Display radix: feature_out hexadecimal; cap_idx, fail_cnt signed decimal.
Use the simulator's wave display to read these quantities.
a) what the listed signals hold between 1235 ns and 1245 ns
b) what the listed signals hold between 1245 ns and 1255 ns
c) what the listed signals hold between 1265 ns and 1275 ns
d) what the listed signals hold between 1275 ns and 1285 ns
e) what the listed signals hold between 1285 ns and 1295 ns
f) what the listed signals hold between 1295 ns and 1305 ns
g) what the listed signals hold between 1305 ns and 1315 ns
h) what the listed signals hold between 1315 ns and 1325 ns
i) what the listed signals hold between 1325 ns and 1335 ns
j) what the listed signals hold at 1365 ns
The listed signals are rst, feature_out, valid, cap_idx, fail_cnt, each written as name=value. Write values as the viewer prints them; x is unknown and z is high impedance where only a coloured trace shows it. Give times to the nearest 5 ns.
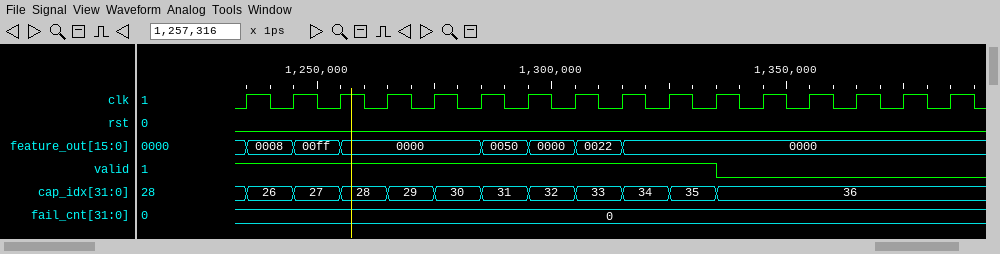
rst=0, feature_out=0008, valid=1, cap_idx=26, fail_cnt=0
rst=0, feature_out=00ff, valid=1, cap_idx=27, fail_cnt=0
rst=0, feature_out=0000, valid=1, cap_idx=29, fail_cnt=0
rst=0, feature_out=0000, valid=1, cap_idx=30, fail_cnt=0
rst=0, feature_out=0050, valid=1, cap_idx=31, fail_cnt=0
rst=0, feature_out=0000, valid=1, cap_idx=32, fail_cnt=0
rst=0, feature_out=0022, valid=1, cap_idx=33, fail_cnt=0
rst=0, feature_out=0000, valid=1, cap_idx=34, fail_cnt=0
rst=0, feature_out=0000, valid=1, cap_idx=35, fail_cnt=0
rst=0, feature_out=0000, valid=0, cap_idx=36, fail_cnt=0
